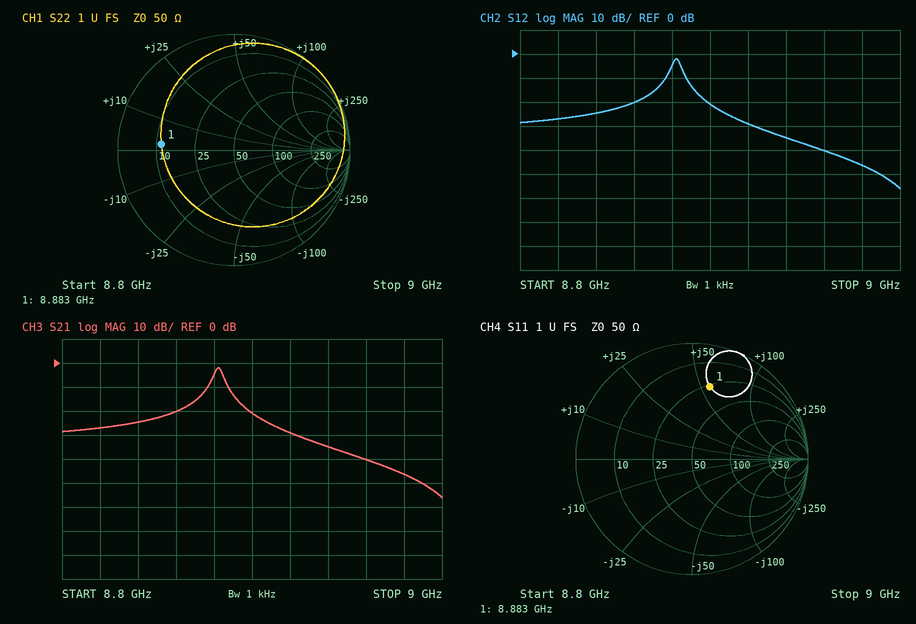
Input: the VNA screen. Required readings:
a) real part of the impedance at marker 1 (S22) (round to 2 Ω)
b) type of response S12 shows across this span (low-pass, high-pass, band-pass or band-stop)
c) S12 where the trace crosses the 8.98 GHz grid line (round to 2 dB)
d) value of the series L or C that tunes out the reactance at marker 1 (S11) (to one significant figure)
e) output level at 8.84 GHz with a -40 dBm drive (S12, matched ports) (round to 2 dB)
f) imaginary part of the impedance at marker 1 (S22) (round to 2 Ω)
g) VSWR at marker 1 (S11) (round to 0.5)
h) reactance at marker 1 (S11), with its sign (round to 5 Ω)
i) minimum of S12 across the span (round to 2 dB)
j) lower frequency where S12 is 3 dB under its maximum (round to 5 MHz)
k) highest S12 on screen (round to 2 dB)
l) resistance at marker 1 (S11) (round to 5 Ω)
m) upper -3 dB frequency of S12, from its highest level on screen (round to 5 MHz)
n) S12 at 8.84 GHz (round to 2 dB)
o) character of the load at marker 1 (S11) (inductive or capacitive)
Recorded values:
12 Ω
band-pass
-46 dB
300 fF
-64 dBm
+2 Ω
4.5
+55 Ω
-56 dB
8.880 GHz
-2 dB
25 Ω
8.885 GHz
-24 dB
inductive
